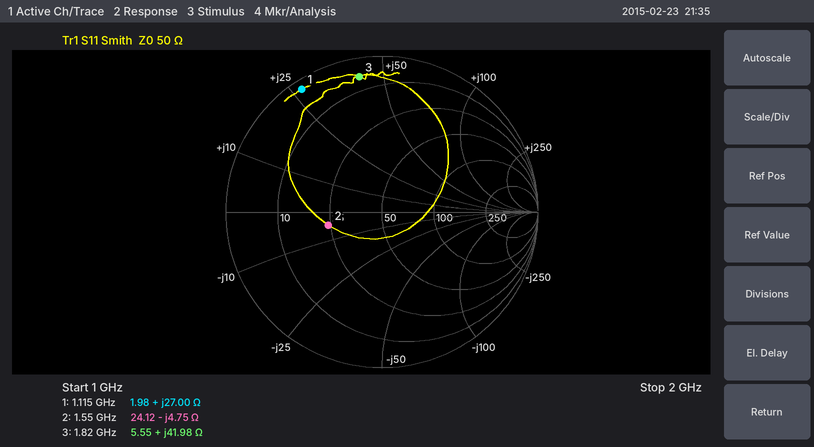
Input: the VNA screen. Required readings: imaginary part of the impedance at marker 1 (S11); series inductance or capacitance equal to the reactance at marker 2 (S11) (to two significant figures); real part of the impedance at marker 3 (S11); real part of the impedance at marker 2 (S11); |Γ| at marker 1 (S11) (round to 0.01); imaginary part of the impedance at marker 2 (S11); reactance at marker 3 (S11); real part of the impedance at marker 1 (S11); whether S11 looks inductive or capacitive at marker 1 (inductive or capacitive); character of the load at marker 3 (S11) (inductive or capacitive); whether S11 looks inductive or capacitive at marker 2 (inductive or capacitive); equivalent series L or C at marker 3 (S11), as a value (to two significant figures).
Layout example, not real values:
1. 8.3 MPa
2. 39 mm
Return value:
1. +27.00 Ω
2. 22 pF
3. 5.55 Ω
4. 24.12 Ω
5. 0.94
6. -4.75 Ω
7. +41.98 Ω
8. 1.98 Ω
9. inductive
10. inductive
11. capacitive
12. 3.7 nH
